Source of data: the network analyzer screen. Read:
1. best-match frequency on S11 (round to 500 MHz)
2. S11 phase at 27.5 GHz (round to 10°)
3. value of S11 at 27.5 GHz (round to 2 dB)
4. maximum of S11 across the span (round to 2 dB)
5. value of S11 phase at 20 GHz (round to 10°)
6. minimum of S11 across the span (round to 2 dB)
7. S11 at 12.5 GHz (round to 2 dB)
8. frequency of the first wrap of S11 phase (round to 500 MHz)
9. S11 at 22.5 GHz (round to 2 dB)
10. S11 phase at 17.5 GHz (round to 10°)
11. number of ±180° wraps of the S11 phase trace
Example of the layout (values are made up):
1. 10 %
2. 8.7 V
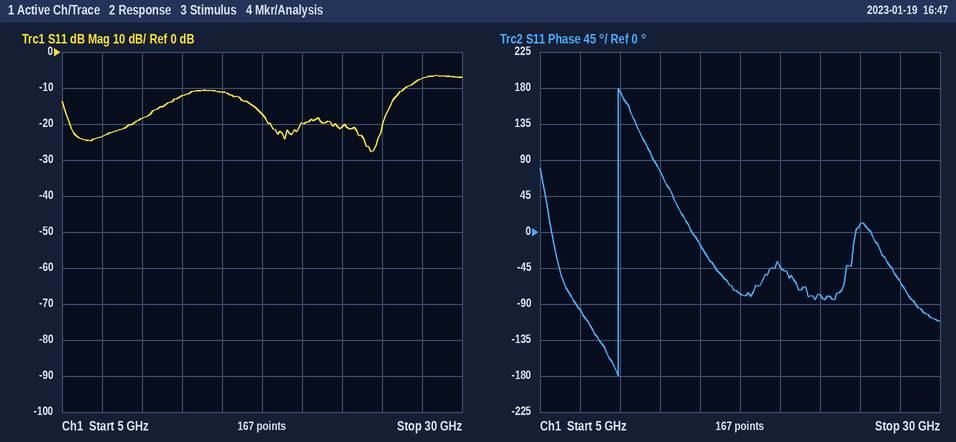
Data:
1. 24.5 GHz
2. -60°
3. -8 dB
4. -6 dB
5. -40°
6. -28 dB
7. -12 dB
8. 10.0 GHz
9. -20 dB
10. -80°
11. 1
